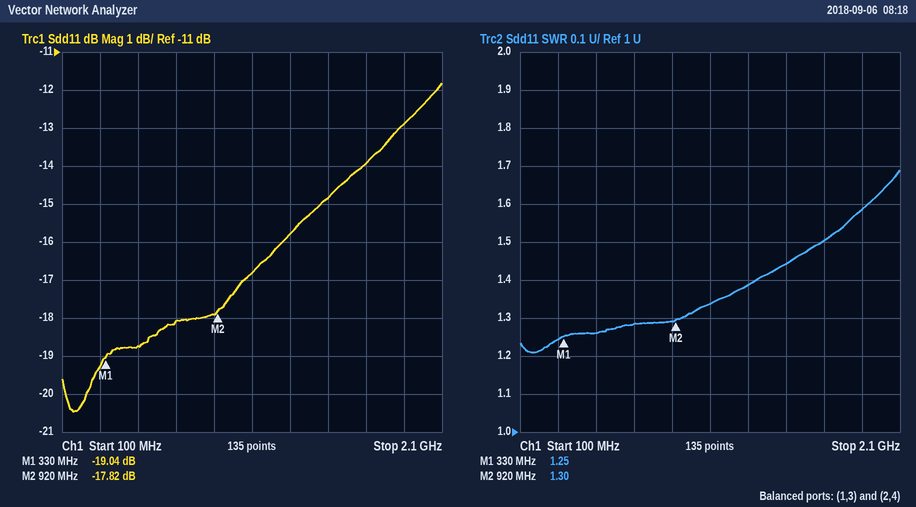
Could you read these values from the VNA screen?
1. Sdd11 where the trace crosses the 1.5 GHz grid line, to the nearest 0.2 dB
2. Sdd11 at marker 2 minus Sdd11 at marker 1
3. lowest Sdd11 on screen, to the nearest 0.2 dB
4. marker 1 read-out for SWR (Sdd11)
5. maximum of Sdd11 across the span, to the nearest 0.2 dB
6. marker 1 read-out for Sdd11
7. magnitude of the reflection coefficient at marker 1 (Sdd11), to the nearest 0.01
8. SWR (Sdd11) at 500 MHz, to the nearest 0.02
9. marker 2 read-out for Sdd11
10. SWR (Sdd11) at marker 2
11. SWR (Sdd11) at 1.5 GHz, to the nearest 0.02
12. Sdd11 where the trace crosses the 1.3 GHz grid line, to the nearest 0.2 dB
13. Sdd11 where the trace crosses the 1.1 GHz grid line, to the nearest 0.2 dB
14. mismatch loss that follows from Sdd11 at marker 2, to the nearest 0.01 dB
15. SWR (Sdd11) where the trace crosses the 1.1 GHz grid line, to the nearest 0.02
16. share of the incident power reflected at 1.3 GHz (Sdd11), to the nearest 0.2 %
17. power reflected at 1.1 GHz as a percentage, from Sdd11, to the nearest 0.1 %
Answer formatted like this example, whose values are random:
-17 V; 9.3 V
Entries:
-14.8 dB; 1.22 dB; -20.4 dB; 1.25; -11.8 dB; -19.04 dB; 0.11; 1.26; -17.82 dB; 1.30; 1.44; -15.8 dB; -16.8 dB; 0.07 dB; 1.34; 2.6 %; 2.1 %
